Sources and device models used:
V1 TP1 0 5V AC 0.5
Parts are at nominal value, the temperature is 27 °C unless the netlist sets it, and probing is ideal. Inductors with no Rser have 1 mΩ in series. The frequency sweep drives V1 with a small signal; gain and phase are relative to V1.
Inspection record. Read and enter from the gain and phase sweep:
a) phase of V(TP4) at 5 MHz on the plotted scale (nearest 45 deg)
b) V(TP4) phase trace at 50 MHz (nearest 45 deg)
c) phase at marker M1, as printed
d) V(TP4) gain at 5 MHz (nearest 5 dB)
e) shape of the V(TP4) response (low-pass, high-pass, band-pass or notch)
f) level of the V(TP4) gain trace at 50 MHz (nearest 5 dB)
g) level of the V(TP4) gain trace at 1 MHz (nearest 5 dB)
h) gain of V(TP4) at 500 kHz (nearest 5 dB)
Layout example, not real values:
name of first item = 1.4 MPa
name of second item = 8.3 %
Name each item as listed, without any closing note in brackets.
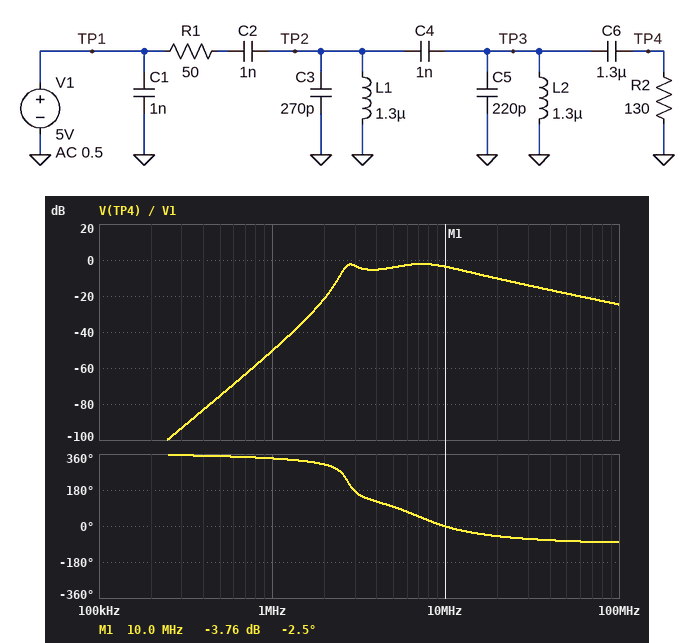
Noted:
phase of V(TP4) at 5 MHz on the plotted scale = 90 deg
V(TP4) phase trace at 50 MHz = -90 deg
phase at marker M1, as printed = -2.5 deg
V(TP4) gain at 5 MHz = -5 dB
shape of the V(TP4) response = band-pass
level of the V(TP4) gain trace at 50 MHz = -20 dB
level of the V(TP4) gain trace at 1 MHz = -50 dB
gain of V(TP4) at 500 kHz = -75 dB
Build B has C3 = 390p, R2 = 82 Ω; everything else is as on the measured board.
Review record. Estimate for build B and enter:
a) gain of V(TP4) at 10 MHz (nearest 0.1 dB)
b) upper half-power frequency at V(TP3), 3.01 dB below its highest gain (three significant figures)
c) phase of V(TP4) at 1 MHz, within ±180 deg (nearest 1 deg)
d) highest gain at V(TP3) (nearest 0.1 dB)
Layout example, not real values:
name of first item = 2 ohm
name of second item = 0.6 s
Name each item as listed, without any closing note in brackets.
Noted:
gain of V(TP4) at 10 MHz = -6.0 dB
upper half-power frequency at V(TP3), 3.01 dB below its highest gain = 11.0 MHz
phase of V(TP4) at 1 MHz, within ±180 deg = -24 deg
highest gain at V(TP3) = -3.9 dB
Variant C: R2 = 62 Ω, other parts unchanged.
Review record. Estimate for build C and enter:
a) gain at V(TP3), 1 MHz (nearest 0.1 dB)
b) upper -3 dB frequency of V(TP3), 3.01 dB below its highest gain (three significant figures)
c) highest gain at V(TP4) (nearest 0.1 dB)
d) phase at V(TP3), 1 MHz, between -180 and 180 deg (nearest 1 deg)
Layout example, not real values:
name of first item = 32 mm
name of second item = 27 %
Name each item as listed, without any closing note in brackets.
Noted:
gain at V(TP3), 1 MHz = -50.5 dB
upper -3 dB frequency of V(TP3), 3.01 dB below its highest gain = 13.9 MHz
highest gain at V(TP4) = -5.1 dB
phase at V(TP3), 1 MHz, between -180 and 180 deg = -26 deg
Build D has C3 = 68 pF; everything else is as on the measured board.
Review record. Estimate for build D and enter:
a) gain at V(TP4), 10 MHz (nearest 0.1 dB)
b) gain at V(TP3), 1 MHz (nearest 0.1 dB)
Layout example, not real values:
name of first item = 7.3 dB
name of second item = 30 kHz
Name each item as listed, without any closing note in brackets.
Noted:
gain at V(TP4), 10 MHz = -2.8 dB
gain at V(TP3), 1 MHz = -50.5 dB
